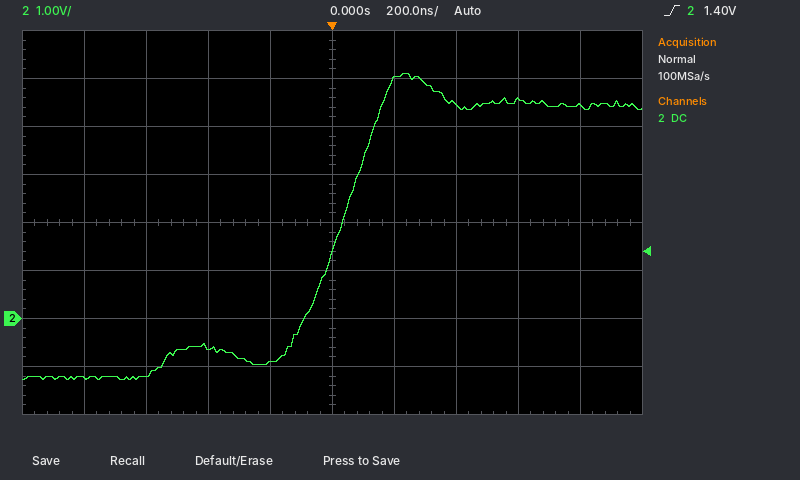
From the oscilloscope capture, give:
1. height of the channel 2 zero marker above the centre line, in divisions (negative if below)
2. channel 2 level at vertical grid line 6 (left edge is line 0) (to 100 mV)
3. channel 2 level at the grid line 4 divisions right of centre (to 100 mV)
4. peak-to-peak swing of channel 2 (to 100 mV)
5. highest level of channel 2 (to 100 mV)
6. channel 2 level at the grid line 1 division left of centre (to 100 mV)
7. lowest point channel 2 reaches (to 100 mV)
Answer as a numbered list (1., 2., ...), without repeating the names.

1. -2.0 div
2. 5.0 V
3. 4.4 V
4. 6.4 V
5. 5.1 V
6. -900 mV
7. -1.3 V
